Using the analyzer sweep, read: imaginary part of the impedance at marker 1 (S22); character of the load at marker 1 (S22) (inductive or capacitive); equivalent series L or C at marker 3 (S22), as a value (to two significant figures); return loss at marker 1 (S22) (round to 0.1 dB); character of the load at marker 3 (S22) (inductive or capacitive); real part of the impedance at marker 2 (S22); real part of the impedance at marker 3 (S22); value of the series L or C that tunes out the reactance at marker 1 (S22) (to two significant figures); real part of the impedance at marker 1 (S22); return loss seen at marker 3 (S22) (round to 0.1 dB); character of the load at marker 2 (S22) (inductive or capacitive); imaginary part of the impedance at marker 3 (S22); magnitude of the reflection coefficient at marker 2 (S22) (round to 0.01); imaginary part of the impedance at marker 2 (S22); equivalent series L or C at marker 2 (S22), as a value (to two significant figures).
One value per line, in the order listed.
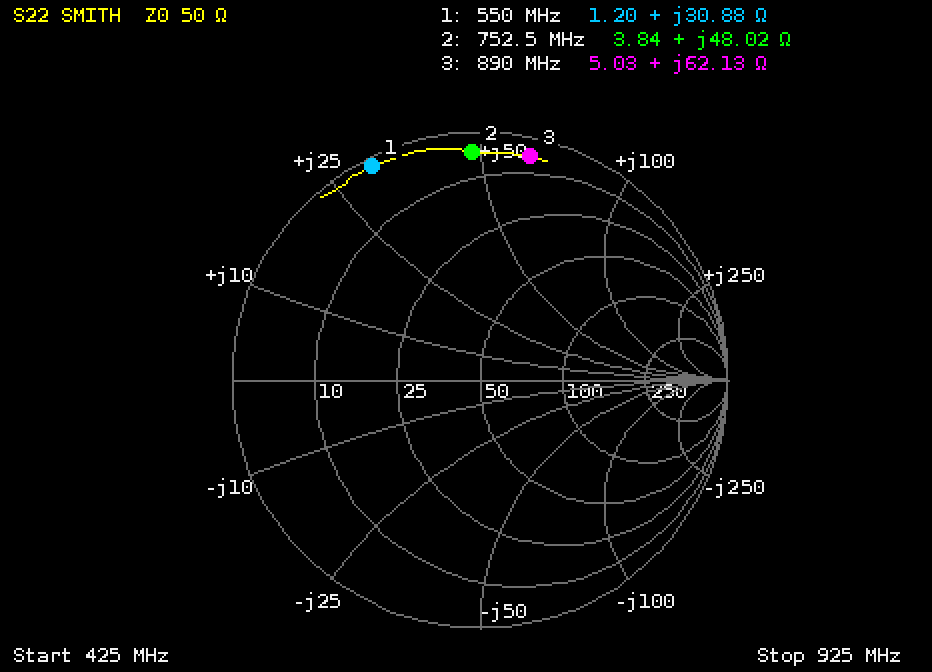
+30.88 Ω
inductive
11 nH
0.3 dB
inductive
3.84 Ω
5.03 Ω
9.4 pF
1.20 Ω
0.7 dB
inductive
+62.13 Ω
0.92
+48.02 Ω
10 nH
